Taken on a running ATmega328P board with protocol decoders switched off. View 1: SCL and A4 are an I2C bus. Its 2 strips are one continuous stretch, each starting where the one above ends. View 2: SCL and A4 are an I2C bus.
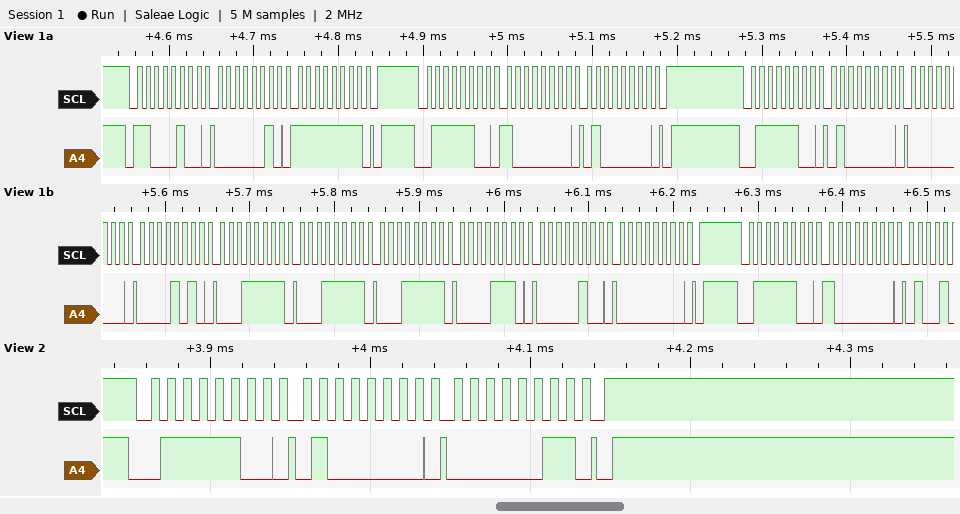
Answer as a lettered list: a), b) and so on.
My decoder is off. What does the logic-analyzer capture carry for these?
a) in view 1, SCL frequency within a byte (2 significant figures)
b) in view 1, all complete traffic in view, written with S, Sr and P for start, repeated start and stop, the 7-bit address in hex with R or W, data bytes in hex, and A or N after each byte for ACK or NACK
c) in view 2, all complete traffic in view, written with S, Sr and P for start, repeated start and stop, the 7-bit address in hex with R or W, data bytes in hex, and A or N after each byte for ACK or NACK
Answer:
a) 100 kHz
b) S 62W A 02 A FF A P S 3EW A 80 A 40 A P S 3EW A 40 A 00 A 0A A 1F A 1F A 1F A 0E A 04 A 00 A P S 3EW A 80 A
c) S 3EW A 40 A 03 A P
